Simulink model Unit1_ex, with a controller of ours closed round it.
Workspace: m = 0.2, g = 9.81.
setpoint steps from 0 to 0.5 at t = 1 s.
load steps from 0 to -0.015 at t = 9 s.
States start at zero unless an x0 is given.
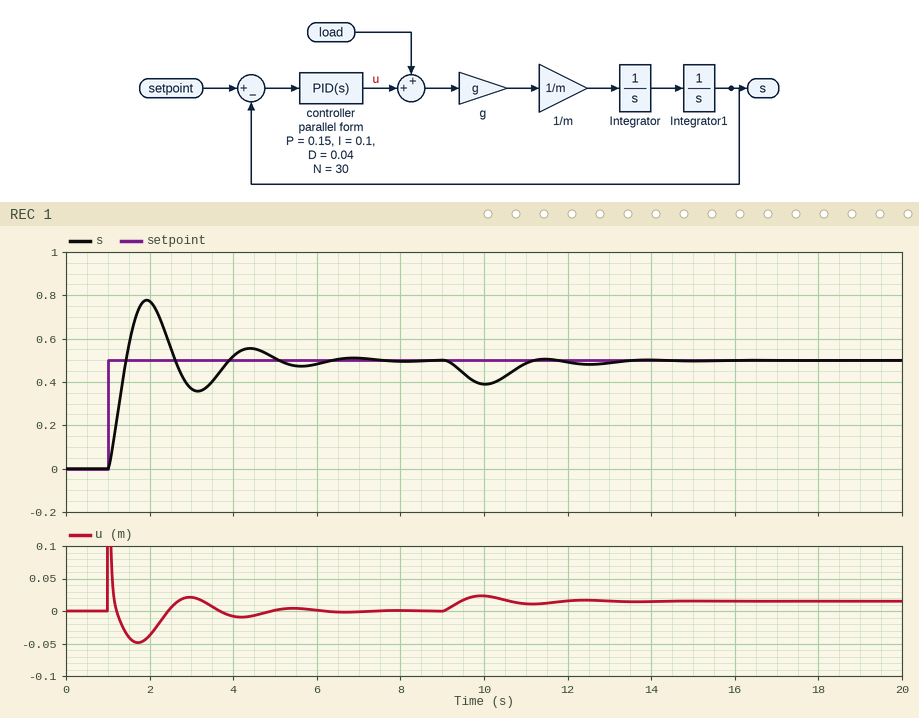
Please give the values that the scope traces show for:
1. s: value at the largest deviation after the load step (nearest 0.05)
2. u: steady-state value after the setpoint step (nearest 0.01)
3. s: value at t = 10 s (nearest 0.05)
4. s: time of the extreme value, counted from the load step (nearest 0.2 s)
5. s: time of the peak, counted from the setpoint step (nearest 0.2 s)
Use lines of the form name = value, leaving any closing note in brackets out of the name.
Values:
s: value at the largest deviation after the load step = 0.40
u: steady-state value after the setpoint step = 0.00
s: value at t = 10 s = 0.40
s: time of the extreme value, counted from the load step = 1.0 s
s: time of the peak, counted from the setpoint step = 1.0 s
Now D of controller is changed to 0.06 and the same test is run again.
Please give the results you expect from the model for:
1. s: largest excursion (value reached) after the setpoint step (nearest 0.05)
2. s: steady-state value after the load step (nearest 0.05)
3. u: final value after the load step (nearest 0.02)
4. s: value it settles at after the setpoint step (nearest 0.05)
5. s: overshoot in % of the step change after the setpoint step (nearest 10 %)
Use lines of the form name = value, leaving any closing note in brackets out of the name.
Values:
s: largest excursion (value reached) after the setpoint step = 0.70
s: steady-state value after the load step = 0.50
u: final value after the load step = 0.02
s: value it settles at after the setpoint step = 0.50
s: overshoot in % of the step change after the setpoint step = 40 %
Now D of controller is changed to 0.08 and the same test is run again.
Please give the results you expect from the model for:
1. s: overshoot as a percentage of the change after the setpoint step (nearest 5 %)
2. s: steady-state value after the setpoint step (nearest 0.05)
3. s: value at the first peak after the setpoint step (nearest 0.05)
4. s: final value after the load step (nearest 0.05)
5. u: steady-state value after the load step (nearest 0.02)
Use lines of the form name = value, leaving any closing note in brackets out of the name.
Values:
s: overshoot as a percentage of the change after the setpoint step = 30 %
s: steady-state value after the setpoint step = 0.50
s: value at the first peak after the setpoint step = 0.65
s: final value after the load step = 0.50
u: steady-state value after the load step = 0.02
